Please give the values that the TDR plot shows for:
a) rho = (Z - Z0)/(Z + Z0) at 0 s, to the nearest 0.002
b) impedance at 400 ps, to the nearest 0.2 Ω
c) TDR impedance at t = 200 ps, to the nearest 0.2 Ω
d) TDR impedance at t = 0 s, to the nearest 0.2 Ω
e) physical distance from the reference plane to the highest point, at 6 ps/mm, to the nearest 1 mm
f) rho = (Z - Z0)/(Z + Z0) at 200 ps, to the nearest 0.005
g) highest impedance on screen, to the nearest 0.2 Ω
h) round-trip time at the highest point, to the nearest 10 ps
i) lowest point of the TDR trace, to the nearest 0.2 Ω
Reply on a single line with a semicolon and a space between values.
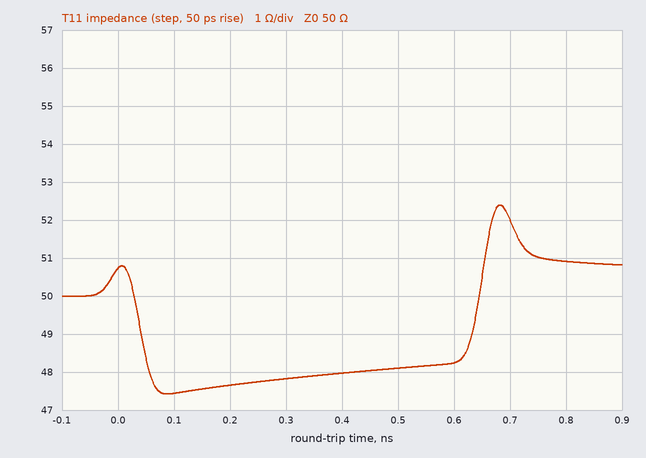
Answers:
+0.008; 48.0 Ω; 47.6 Ω; 50.8 Ω; 57 mm; -0.025; 52.4 Ω; 680 ps; 47.4 Ω
